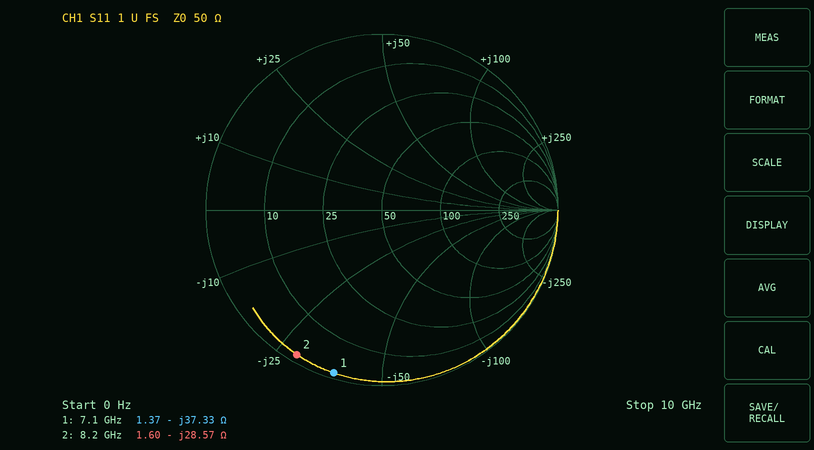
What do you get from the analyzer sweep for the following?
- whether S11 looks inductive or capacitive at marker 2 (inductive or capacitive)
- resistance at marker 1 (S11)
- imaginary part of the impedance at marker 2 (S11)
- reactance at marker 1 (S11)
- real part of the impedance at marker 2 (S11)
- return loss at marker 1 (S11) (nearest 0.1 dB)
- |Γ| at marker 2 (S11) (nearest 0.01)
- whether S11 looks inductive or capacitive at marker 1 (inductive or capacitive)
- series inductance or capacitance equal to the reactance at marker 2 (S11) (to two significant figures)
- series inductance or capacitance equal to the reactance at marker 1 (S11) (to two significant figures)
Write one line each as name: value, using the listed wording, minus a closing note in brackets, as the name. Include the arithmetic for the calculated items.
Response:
whether S11 looks inductive or capacitive at marker 2: capacitive
resistance at marker 1: 1.37 Ω
imaginary part of the impedance at marker 2: -28.57 Ω
reactance at marker 1: -37.33 Ω
real part of the impedance at marker 2: 1.60 Ω
return loss at marker 1 (S11): 0.3 dB
|Γ| at marker 2 (S11): 0.95
whether S11 looks inductive or capacitive at marker 1: capacitive
series inductance or capacitance equal to the reactance at marker 2 (S11): C = 1/(2π × 8.2 GHz × 28.57 Ω) ≈ 679 fF, so 680 fF to two significant figures
series inductance or capacitance equal to the reactance at marker 1 (S11): C = 1/(2π × 7.1 GHz × 37.33 Ω) ≈ 600 fF
